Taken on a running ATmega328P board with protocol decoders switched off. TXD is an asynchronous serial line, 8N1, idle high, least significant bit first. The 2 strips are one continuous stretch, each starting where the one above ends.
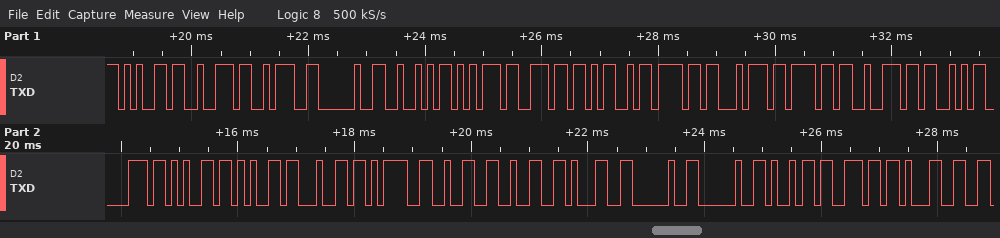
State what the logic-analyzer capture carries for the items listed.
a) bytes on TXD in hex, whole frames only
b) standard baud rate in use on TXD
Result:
65 72 3A 20 52 75 6E 4D 6F 74 6F 72 53 70 65 65 64 3D 32 32 31 20 20 69 6E 31
9600 baud
